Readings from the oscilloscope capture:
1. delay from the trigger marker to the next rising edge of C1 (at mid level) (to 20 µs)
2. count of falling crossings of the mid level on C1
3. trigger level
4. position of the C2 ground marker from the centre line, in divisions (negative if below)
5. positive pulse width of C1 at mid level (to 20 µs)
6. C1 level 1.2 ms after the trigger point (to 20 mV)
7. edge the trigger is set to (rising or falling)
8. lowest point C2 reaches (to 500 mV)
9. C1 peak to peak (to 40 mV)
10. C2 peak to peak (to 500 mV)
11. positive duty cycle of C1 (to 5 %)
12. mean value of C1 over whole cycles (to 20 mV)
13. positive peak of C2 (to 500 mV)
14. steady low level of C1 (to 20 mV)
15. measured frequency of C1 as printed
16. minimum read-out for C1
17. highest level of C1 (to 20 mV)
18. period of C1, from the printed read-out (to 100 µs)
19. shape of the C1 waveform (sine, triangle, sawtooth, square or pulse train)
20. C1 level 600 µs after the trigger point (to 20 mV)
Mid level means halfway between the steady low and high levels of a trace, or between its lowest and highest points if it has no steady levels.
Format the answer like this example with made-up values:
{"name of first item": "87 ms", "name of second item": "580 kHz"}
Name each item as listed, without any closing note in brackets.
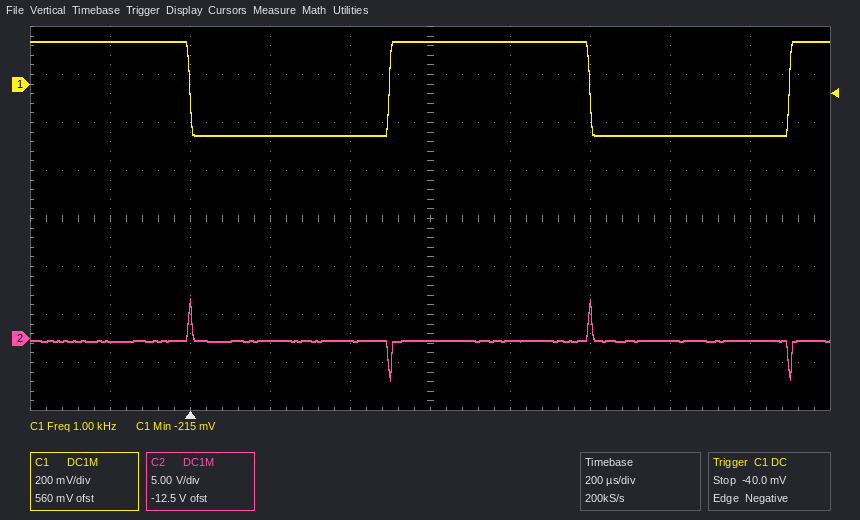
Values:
{"delay from the trigger marker to the next rising edge of C1 (at mid level)": "500 µs", "count of falling crossings of the mid level on C1": "2", "trigger level": "-40.0 mV", "position of the C2 ground marker from the centre line, in divisions": "-2.5 div", "positive pulse width of C1 at mid level": "500 µs", "C1 level 1.2 ms after the trigger point": "-220 mV", "edge the trigger is set to": "falling", "lowest point C2 reaches": "-4.5 V", "C1 peak to peak": "400 mV", "C2 peak to peak": "8.5 V", "positive duty cycle of C1": "50 %", "mean value of C1 over whole cycles": "-20 mV", "positive peak of C2": "4.0 V", "steady low level of C1": "-220 mV", "measured frequency of C1 as printed": "1.00 kHz", "minimum read-out for C1": "-215 mV", "highest level of C1": "180 mV", "period of C1, from the printed read-out": "1.0 ms", "shape of the C1 waveform": "square", "C1 level 600 µs after the trigger point": "180 mV"}
